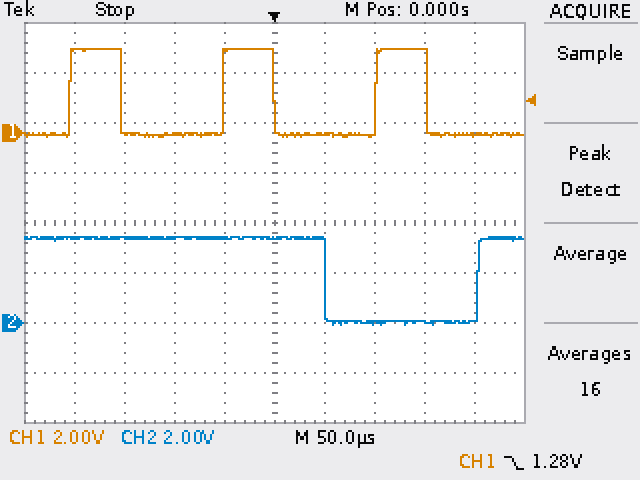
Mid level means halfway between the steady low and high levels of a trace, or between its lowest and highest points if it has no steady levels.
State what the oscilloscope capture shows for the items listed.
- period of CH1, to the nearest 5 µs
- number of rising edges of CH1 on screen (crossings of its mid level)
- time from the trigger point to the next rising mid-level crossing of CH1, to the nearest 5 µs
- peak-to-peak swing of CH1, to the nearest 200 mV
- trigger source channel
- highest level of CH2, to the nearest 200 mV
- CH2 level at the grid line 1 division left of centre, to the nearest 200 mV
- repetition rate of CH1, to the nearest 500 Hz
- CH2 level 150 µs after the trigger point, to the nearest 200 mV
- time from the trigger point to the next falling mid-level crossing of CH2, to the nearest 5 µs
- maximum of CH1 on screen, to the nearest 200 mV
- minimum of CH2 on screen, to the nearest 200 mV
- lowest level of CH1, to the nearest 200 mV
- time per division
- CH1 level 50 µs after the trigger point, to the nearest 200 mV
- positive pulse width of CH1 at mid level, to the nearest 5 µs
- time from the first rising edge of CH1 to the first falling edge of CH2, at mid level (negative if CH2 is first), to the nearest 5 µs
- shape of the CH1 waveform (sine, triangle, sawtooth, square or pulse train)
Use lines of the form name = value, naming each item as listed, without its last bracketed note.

period of CH1, to the nearest 5 µs = 155 µs
number of rising edges of CH1 on screen = 3
time from the trigger point to the next rising mid-level crossing of CH1, to the nearest 5 µs = 100 µs
peak-to-peak swing of CH1, to the nearest 200 mV = 3.6 V
trigger source channel = CH1
highest level of CH2, to the nearest 200 mV = 3.4 V
CH2 level at the grid line 1 division left of centre, to the nearest 200 mV = 3.4 V
repetition rate of CH1, to the nearest 500 Hz = 6.5 kHz
CH2 level 150 µs after the trigger point, to the nearest 200 mV = 0.0 V
time from the trigger point to the next falling mid-level crossing of CH2, to the nearest 5 µs = 50 µs
maximum of CH1 on screen, to the nearest 200 mV = 3.4 V
minimum of CH2 on screen, to the nearest 200 mV = 0.0 V
lowest level of CH1, to the nearest 200 mV = -200 mV
time per division = 50 µs
CH1 level 50 µs after the trigger point, to the nearest 200 mV = 0.0 V
positive pulse width of CH1 at mid level, to the nearest 5 µs = 50 µs
time from the first rising edge of CH1 to the first falling edge of CH2, at mid level (negative if CH2 is first), to the nearest 5 µs = +255 µs
shape of the CH1 waveform = pulse train
